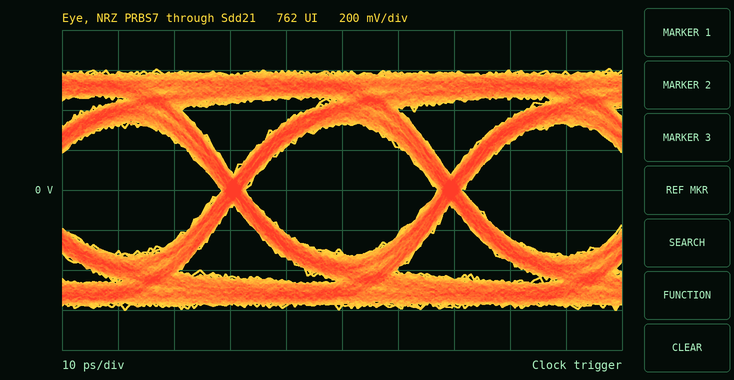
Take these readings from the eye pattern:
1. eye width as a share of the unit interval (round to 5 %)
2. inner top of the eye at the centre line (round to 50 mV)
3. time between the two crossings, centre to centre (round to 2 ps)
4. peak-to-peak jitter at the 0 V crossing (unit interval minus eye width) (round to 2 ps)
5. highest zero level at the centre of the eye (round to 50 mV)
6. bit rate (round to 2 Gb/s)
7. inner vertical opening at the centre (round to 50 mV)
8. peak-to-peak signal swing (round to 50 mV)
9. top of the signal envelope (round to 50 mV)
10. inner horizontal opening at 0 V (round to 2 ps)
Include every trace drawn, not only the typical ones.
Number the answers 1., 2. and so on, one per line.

1. 90 %
2. 350 mV
3. 38 ps
4. 4 ps
5. -300 mV
6. 26 Gb/s
7. 650 mV
8. 1.20 V
9. 600 mV
10. 34 ps
